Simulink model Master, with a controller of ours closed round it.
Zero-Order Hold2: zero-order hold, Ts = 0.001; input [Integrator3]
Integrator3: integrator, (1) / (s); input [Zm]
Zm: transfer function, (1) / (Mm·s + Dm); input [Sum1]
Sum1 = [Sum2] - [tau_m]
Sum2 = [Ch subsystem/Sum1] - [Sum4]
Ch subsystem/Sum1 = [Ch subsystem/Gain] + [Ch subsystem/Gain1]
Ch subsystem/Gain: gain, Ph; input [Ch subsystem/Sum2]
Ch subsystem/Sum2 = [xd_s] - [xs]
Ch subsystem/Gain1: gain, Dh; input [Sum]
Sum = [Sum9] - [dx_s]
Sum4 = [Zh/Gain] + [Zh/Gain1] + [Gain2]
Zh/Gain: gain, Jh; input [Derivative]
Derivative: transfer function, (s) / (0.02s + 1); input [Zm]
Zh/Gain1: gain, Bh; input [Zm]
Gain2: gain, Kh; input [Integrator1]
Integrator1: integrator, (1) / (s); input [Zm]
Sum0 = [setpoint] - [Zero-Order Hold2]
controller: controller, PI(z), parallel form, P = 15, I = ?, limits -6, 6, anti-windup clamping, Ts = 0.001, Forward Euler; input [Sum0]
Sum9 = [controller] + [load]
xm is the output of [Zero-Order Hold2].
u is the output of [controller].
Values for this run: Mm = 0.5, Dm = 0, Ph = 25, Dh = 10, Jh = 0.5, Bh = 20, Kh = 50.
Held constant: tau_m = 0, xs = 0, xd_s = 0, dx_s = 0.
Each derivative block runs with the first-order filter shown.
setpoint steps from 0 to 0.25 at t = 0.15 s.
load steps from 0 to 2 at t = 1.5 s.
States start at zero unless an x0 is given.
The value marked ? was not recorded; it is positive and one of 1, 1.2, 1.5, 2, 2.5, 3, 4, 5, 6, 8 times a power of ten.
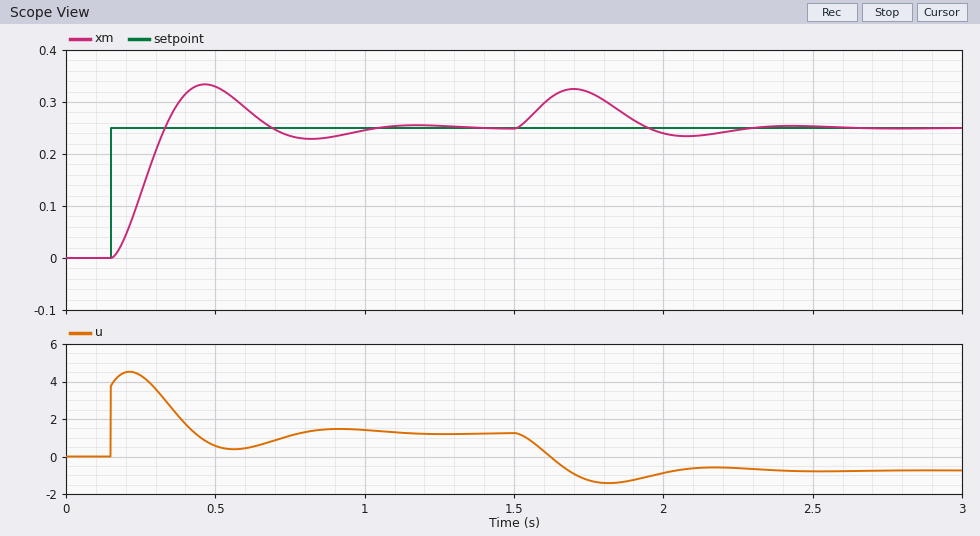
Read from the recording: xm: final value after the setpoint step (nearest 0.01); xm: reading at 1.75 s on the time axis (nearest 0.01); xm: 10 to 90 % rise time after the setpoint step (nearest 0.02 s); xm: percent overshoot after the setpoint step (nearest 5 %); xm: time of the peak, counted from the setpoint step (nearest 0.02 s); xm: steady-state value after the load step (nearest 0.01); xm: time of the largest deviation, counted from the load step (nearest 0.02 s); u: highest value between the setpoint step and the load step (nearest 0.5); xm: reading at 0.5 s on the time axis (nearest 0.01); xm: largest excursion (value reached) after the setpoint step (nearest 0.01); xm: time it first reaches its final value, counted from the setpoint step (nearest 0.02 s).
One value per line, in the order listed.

0.25
0.32
0.12 s
35 %
0.32 s
0.25
0.20 s
4.5
0.33
0.33
0.18 s
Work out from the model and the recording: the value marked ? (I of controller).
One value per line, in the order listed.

120
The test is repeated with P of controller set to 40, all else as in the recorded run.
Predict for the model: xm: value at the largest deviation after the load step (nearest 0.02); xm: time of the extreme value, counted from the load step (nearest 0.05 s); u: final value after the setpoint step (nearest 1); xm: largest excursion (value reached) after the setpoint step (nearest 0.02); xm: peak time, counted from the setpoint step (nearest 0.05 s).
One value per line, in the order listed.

0.30
0.15 s
1
0.26
0.20 s
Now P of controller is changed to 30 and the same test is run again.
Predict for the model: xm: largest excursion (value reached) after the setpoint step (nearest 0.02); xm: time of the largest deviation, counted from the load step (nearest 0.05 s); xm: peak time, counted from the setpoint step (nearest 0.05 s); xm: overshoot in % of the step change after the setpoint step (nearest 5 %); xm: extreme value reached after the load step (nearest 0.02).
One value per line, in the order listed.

0.28
0.15 s
0.25 s
10 %
0.30
